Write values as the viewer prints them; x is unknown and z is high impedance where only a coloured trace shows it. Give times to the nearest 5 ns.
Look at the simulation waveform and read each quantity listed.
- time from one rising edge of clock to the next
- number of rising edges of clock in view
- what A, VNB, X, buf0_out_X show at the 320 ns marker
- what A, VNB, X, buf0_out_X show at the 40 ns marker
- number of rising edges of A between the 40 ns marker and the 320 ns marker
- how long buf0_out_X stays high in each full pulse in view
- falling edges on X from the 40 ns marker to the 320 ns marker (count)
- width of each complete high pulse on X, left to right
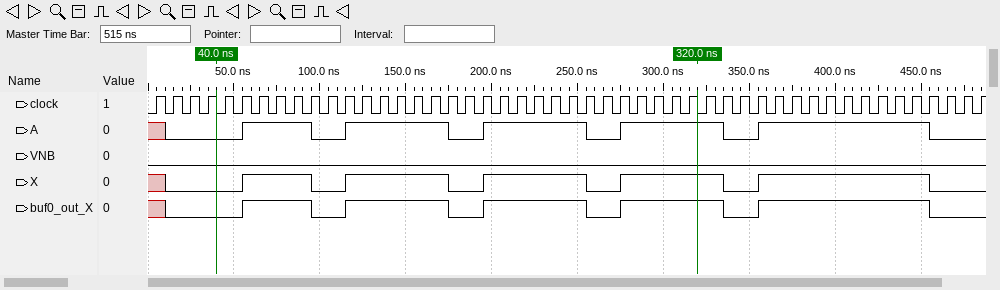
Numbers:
10 ns
49
A=1, VNB=0, X=1, buf0_out_X=1
A=0, VNB=0, X=0, buf0_out_X=0
4
40 ns, 60 ns, 60 ns, 60 ns, 100 ns
3
40 ns, 60 ns, 60 ns, 60 ns, 100 ns
